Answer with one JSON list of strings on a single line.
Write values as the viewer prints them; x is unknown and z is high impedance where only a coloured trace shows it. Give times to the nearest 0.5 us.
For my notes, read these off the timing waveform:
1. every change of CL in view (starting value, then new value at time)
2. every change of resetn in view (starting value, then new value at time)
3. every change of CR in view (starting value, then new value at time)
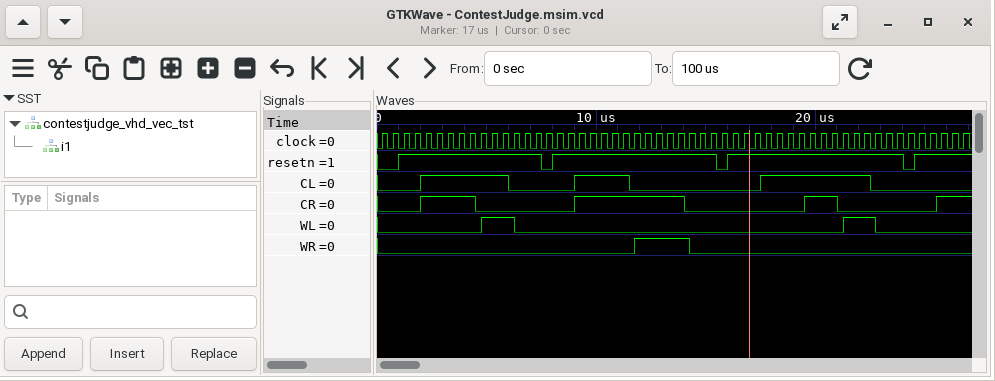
["0, 1 at 2 us, 0 at 6 us, 1 at 9 us, 0 at 11.5 us, 1 at 17.5 us, 0 at 22.5 us", "0, 1 at 1 us, 0 at 7.5 us, 1 at 8 us, 0 at 15.5 us, 1 at 16 us, 0 at 24 us, 1 at 24.5 us", "0, 1 at 2 us, 0 at 4.5 us, 1 at 9 us, 0 at 14 us, 1 at 19.5 us, 0 at 21 us, 1 at 25.5 us"]
